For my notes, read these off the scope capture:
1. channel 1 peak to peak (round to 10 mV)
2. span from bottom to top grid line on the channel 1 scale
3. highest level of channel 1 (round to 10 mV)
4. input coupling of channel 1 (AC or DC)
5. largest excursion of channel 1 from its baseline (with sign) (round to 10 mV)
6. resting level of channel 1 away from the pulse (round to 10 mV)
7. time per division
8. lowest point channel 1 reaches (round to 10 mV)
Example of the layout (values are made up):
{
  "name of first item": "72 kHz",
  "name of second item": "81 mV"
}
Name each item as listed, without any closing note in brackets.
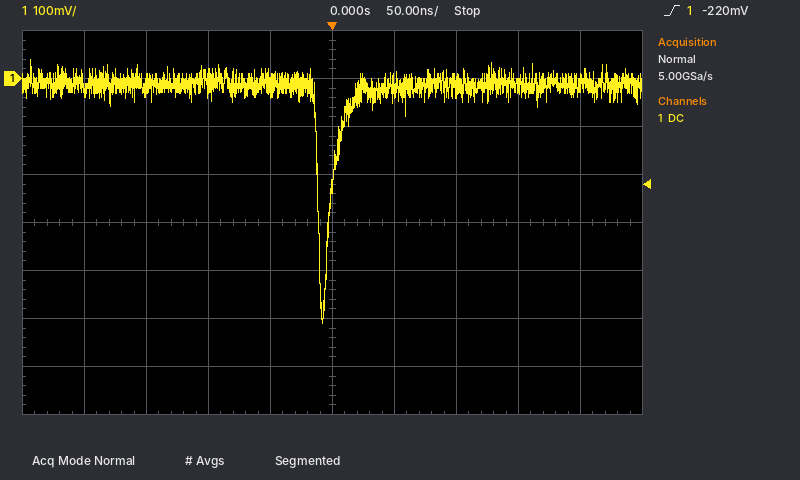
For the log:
{
  "channel 1 peak to peak": "550 mV",
  "span from bottom to top grid line on the channel 1 scale": "800 mV",
  "highest level of channel 1": "40 mV",
  "input coupling of channel 1": "DC",
  "largest excursion of channel 1 from its baseline (with sign)": "-500 mV",
  "resting level of channel 1 away from the pulse": "-10 mV",
  "time per division": "50 ns",
  "lowest point channel 1 reaches": "-510 mV"
}
